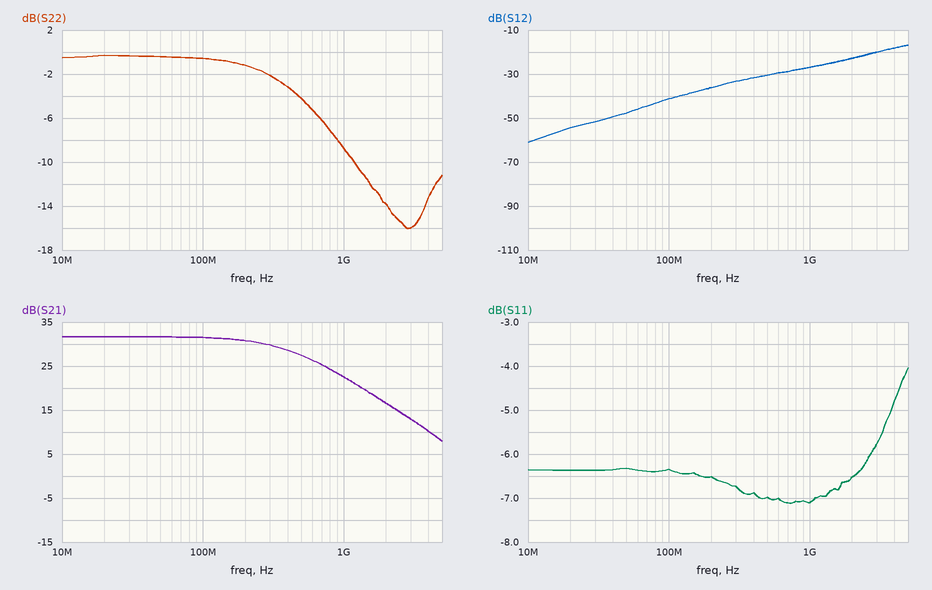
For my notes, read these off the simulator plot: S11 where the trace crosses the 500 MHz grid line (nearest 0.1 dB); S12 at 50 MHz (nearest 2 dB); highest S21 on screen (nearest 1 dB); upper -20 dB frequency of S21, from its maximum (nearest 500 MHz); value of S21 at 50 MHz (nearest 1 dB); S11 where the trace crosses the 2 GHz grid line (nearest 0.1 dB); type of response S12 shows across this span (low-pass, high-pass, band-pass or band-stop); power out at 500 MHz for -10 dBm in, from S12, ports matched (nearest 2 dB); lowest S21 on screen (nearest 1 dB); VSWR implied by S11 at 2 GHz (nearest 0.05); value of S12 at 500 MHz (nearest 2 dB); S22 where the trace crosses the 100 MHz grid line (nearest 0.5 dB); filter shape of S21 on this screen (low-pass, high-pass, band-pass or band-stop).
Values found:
-7.0 dB
-48 dB
32 dB
3.5 GHz
32 dB
-6.5 dB
high-pass
-40 dBm
8 dB
2.80
-30 dB
-0.5 dB
low-pass
